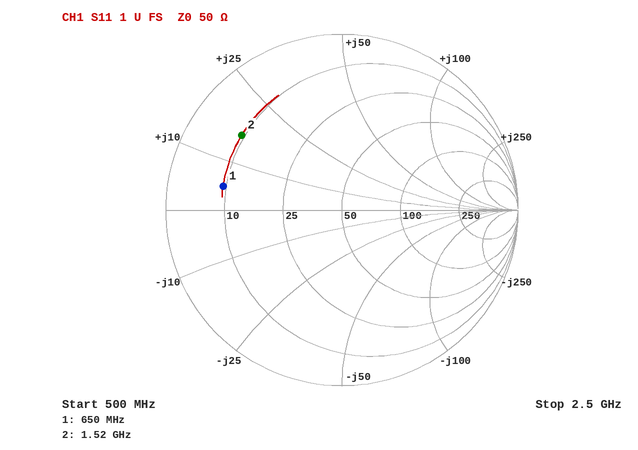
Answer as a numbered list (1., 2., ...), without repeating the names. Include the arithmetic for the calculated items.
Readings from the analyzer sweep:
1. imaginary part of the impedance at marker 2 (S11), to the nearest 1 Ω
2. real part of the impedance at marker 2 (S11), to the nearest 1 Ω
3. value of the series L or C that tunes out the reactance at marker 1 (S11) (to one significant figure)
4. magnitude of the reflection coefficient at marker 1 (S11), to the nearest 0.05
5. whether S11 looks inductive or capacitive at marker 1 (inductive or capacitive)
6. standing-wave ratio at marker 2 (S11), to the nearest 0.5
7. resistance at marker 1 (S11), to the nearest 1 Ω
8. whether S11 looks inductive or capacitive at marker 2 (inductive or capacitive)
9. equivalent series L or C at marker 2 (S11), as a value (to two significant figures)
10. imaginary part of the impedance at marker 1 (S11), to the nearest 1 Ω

1. +16 Ω
2. 9 Ω
3. C = 1/(2π × 650 MHz × 5 Ω) ≈ 49.0 pF, so 50 pF to one significant figure
4. 0.70
5. inductive
6. 6.0
7. 9 Ω
8. inductive
9. L = 16 Ω/(2π × 1.52 GHz) ≈ 1.7 nH
10. +5 Ω
